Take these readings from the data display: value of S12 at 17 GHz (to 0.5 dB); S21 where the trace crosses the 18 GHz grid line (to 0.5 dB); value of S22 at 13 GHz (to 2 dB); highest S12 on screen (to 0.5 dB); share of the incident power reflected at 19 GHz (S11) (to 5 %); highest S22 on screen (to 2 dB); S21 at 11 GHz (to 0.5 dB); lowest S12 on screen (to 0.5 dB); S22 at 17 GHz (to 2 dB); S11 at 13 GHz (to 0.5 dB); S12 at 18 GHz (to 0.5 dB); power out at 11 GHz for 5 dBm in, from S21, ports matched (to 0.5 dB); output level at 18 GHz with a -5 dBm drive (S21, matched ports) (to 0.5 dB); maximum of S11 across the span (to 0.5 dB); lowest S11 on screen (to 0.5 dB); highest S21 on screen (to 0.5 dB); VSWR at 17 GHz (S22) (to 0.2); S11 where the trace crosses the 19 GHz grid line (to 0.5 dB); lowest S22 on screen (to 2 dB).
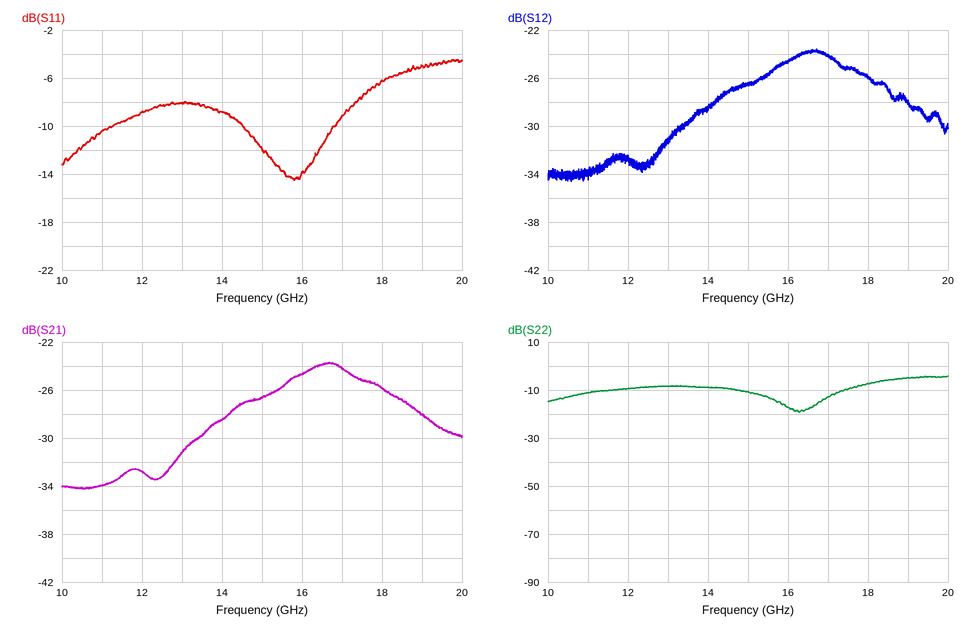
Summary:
-24.0 dB
-26.0 dB
-8 dB
-23.5 dB
30 %
-4 dB
-34.0 dB
-34.5 dB
-12 dB
-8.0 dB
-26.0 dB
-29.0 dBm
-31.0 dBm
-4.5 dB
-14.5 dB
-23.5 dB
1.6
-5.0 dB
-20 dB
